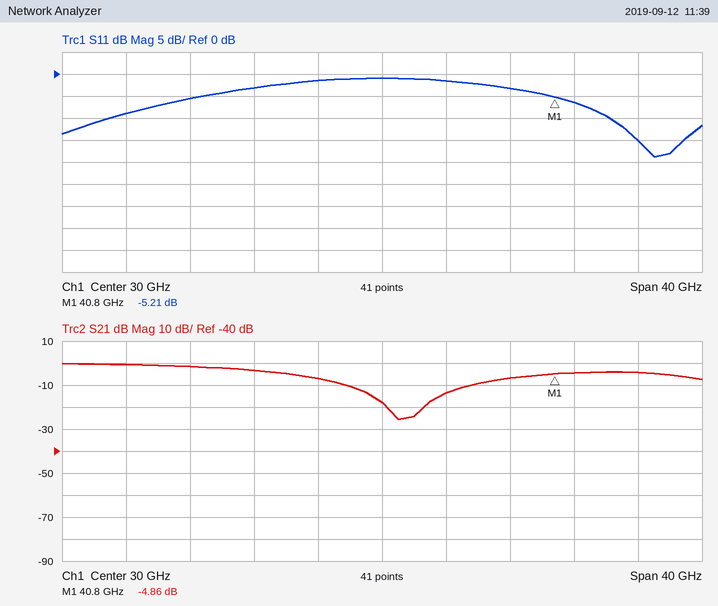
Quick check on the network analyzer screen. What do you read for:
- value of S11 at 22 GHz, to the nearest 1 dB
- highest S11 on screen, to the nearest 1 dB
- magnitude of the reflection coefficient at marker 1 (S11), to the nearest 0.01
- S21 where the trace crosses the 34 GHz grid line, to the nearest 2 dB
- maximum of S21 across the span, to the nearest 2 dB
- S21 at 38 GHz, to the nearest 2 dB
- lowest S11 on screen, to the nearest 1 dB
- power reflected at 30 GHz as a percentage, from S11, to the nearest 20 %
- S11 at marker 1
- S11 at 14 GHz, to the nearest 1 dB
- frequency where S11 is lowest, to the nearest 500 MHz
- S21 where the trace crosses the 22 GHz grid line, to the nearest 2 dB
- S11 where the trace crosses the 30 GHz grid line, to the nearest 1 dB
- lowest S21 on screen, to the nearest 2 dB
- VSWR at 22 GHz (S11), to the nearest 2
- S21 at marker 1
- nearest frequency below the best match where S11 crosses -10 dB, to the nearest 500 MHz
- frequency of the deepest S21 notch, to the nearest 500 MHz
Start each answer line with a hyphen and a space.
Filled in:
- -3 dB
- -1 dB
- 0.55
- -14 dB
- 0 dB
- -6 dB
- -19 dB
- 80 %
- -5.21 dB
- -9 dB
- 47.0 GHz
- -4 dB
- -1 dB
- -26 dB
- 6
- -4.86 dB
- 44.0 GHz
- 31.0 GHz
